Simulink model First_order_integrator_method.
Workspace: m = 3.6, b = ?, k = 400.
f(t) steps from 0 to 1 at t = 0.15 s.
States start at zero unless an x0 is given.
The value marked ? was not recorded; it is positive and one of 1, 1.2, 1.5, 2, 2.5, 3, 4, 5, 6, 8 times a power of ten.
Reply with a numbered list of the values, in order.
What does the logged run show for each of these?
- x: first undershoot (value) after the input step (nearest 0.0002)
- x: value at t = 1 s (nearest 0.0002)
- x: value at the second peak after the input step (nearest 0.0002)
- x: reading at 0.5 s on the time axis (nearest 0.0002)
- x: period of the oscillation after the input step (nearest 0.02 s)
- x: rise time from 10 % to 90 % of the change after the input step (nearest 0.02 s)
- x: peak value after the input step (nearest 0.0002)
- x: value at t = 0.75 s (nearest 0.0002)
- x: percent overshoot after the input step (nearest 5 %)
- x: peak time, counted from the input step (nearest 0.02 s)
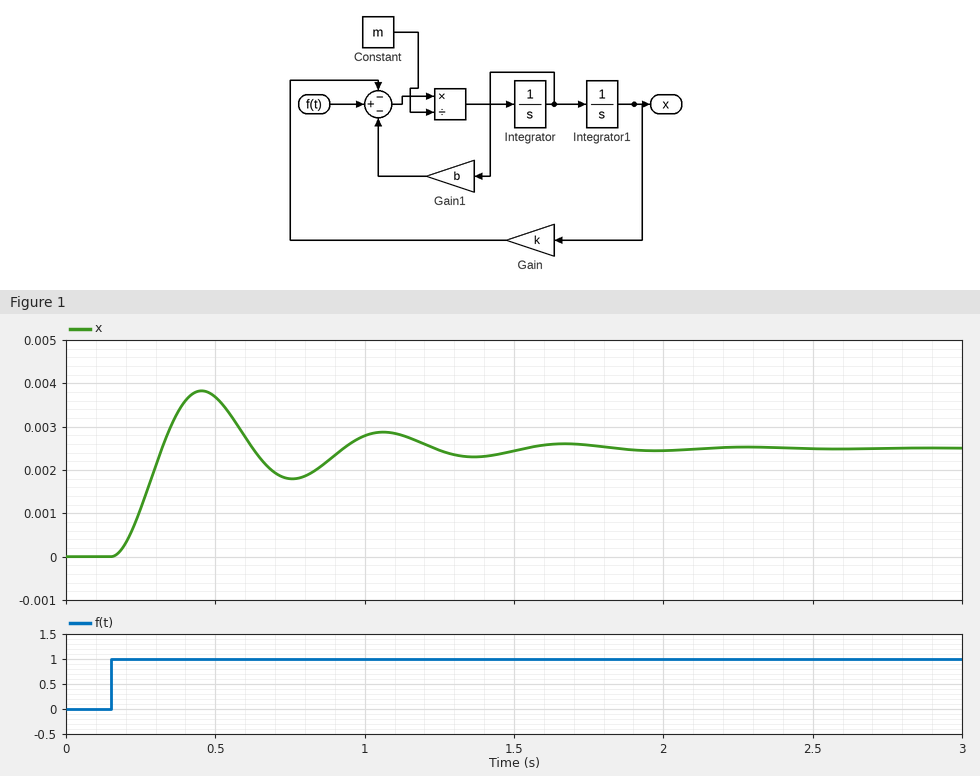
1. 0.0018
2. 0.0028
3. 0.0028
4. 0.0036
5. 0.60 s
6. 0.12 s
7. 0.0038
8. 0.0018
9. 55 %
10. 0.30 s
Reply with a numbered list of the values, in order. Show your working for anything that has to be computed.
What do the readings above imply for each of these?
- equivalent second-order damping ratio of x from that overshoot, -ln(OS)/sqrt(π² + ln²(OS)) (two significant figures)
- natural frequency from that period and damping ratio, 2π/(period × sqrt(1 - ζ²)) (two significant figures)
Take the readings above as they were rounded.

1. ln(0.55) = -0.598; 0.598 / sqrt(9.870 + 0.357) = 0.19
2. 2π / (0.6 × sqrt(1 - 0.19²)) = 11 rad/s
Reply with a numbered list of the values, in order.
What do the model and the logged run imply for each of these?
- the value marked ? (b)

1. 15
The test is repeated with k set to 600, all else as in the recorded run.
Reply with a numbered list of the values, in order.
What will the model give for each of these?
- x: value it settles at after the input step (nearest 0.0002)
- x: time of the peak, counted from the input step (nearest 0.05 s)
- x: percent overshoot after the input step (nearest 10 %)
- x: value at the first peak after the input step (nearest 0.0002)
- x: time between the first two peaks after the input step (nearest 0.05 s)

1. 0.0016
2. 0.25 s
3. 60 %
4. 0.0026
5. 0.50 s
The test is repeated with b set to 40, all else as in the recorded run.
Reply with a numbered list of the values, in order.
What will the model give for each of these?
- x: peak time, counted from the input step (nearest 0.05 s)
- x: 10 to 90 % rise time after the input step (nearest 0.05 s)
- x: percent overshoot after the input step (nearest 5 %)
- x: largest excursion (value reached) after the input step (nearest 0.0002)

1. 0.35 s
2. 0.15 s
3. 15 %
4. 0.0028
